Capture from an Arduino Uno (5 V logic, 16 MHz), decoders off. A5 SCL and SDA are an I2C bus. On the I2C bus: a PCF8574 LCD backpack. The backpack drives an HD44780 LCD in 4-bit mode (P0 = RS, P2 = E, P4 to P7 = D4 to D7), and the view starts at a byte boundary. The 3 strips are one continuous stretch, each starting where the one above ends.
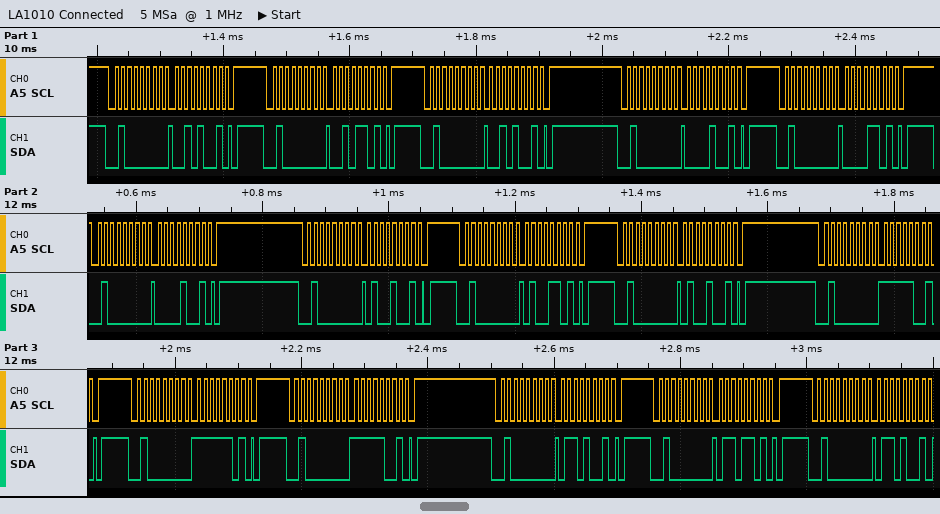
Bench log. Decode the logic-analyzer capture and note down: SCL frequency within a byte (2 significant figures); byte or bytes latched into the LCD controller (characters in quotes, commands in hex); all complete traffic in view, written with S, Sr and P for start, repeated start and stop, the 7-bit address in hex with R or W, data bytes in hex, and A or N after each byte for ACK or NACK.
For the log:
100 kHz
' ' 'O'
S 20W A 29 A P S 20W A 2D A P S 20W A 29 A P S 20W A 09 A P S 20W A 0D A P S 20W A 09 A P S 20W A 49 A P S 20W A 4D A P S 20W A 49 A P S 20W A F9 A P S 20W A FD A P S 20W A F9 A P S 20W A 69 A P S 20W A 6D A P S 20W A 69 A
